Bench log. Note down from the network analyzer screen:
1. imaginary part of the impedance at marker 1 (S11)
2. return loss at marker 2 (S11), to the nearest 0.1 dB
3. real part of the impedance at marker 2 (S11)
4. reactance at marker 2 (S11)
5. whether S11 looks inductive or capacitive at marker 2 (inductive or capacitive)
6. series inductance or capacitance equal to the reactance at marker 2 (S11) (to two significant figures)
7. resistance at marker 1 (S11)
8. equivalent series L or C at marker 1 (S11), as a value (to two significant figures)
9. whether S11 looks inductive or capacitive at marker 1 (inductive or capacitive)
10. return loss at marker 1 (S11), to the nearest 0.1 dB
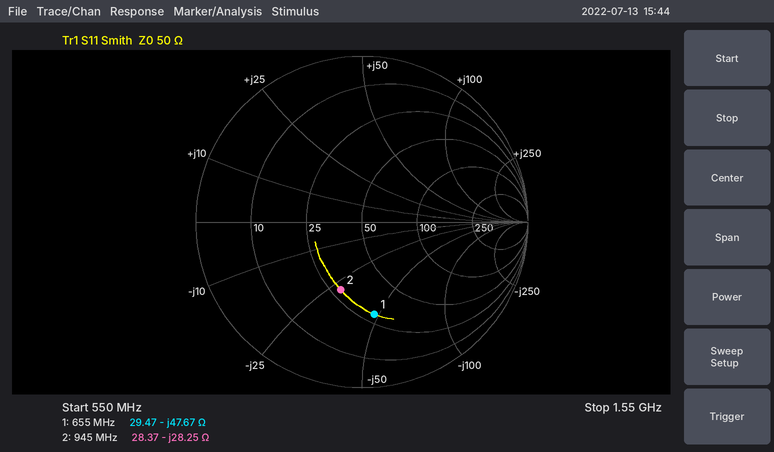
-47.67 Ω
7.4 dB
28.37 Ω
-28.25 Ω
capacitive
6.0 pF
29.47 Ω
5.1 pF
capacitive
5.0 dB
